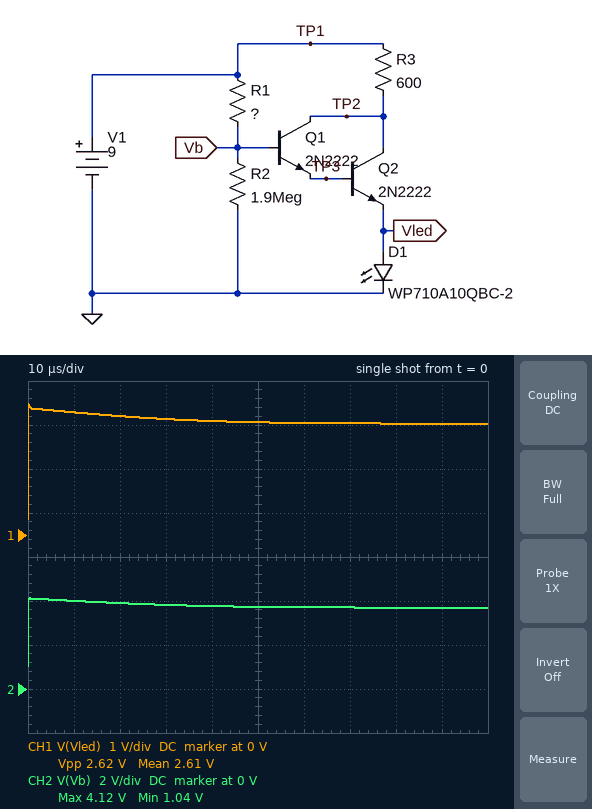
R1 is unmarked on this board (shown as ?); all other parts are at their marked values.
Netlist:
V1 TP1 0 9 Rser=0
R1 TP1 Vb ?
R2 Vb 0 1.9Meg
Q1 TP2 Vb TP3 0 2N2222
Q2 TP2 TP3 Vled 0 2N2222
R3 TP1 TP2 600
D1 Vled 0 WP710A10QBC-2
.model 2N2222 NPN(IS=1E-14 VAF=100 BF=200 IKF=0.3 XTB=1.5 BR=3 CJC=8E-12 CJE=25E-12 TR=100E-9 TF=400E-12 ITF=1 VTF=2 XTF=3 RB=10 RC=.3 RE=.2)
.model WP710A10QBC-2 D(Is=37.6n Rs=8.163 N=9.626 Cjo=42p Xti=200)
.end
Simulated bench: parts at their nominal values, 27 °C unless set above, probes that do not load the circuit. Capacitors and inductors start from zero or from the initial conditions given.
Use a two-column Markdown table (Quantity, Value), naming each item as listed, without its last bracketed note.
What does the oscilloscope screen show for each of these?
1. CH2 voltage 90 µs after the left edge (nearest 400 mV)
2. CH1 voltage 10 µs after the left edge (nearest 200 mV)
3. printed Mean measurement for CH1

| Quantity | Value |
|---|---|
| CH2 voltage 90 µs after the left edge | 3.6 V |
| CH1 voltage 10 µs after the left edge | 2.8 V |
| printed Mean measurement for CH1 | 2.61 V |
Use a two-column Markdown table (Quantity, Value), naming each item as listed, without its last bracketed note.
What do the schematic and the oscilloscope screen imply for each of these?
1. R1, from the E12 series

| Quantity | Value |
|---|---|
| R1, from the E12 series | 2.7 MΩ |
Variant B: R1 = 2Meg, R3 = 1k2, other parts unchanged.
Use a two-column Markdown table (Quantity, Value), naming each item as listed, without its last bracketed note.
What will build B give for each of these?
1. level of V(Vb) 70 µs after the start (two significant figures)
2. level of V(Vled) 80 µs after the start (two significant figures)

| Quantity | Value |
|---|---|
| level of V(Vb) 70 µs after the start | 4.2 V |
| level of V(Vled) 80 µs after the start | 2.9 V |
